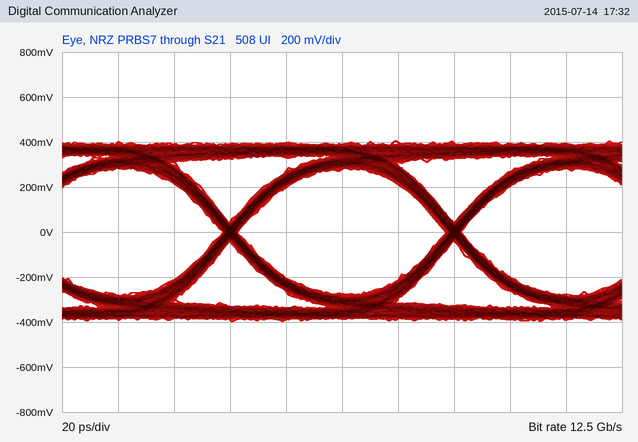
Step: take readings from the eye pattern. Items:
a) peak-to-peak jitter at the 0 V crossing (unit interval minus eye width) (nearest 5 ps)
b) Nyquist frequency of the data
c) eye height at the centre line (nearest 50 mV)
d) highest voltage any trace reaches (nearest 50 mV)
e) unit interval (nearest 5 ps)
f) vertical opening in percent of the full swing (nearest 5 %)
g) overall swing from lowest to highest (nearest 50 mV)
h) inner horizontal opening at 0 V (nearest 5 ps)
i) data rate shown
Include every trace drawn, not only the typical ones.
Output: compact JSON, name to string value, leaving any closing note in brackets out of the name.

{"peak-to-peak jitter at the 0 V crossing (unit interval minus eye width)": "5 ps", "Nyquist frequency of the data": "6.25 GHz", "eye height at the centre line": "550 mV", "highest voltage any trace reaches": "400 mV", "unit interval": "80 ps", "vertical opening in percent of the full swing": "70 %", "overall swing from lowest to highest": "800 mV", "inner horizontal opening at 0 V": "75 ps", "data rate shown": "12.5 Gb/s"}
